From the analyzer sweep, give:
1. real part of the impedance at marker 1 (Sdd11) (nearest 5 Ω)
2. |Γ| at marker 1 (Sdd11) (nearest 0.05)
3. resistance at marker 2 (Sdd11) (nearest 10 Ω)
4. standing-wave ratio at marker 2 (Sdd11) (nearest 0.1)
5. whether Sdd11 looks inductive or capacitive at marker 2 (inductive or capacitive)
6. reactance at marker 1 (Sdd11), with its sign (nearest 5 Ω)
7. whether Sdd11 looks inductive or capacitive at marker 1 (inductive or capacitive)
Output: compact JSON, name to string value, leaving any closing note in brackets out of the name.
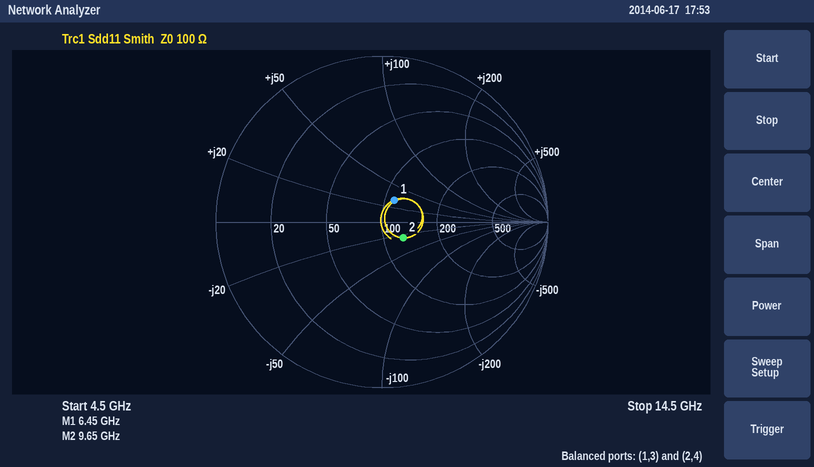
{"real part of the impedance at marker 1 (Sdd11)": "110 Ω", "|Γ| at marker 1 (Sdd11)": "0.15", "resistance at marker 2 (Sdd11)": "130 Ω", "standing-wave ratio at marker 2 (Sdd11)": "1.4", "whether Sdd11 looks inductive or capacitive at marker 2": "capacitive", "reactance at marker 1 (Sdd11), with its sign": "+30 Ω", "whether Sdd11 looks inductive or capacitive at marker 1": "inductive"}
